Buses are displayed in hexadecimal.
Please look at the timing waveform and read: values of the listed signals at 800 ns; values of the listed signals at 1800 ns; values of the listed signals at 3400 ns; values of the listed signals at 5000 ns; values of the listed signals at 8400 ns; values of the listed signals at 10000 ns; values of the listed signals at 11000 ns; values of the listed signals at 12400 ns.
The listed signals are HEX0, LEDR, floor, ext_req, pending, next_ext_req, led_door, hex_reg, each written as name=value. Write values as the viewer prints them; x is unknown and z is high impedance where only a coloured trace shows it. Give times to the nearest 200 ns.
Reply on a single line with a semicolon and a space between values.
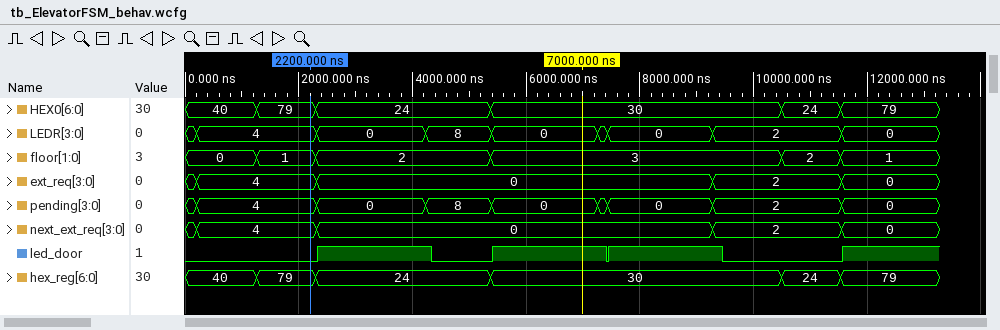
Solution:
HEX0=40, LEDR=4, floor=0, ext_req=4, pending=4, next_ext_req=4, led_door=0, hex_reg=40; HEX0=79, LEDR=4, floor=1, ext_req=4, pending=4, next_ext_req=4, led_door=0, hex_reg=79; HEX0=24, LEDR=0, floor=2, ext_req=0, pending=0, next_ext_req=0, led_door=1, hex_reg=24; HEX0=24, LEDR=8, floor=2, ext_req=0, pending=8, next_ext_req=0, led_door=0, hex_reg=24; HEX0=30, LEDR=0, floor=3, ext_req=0, pending=0, next_ext_req=0, led_door=1, hex_reg=30; HEX0=30, LEDR=2, floor=3, ext_req=2, pending=2, next_ext_req=2, led_door=0, hex_reg=30; HEX0=24, LEDR=2, floor=2, ext_req=2, pending=2, next_ext_req=2, led_door=0, hex_reg=24; HEX0=79, LEDR=0, floor=1, ext_req=0, pending=0, next_ext_req=0, led_door=1, hex_reg=79
